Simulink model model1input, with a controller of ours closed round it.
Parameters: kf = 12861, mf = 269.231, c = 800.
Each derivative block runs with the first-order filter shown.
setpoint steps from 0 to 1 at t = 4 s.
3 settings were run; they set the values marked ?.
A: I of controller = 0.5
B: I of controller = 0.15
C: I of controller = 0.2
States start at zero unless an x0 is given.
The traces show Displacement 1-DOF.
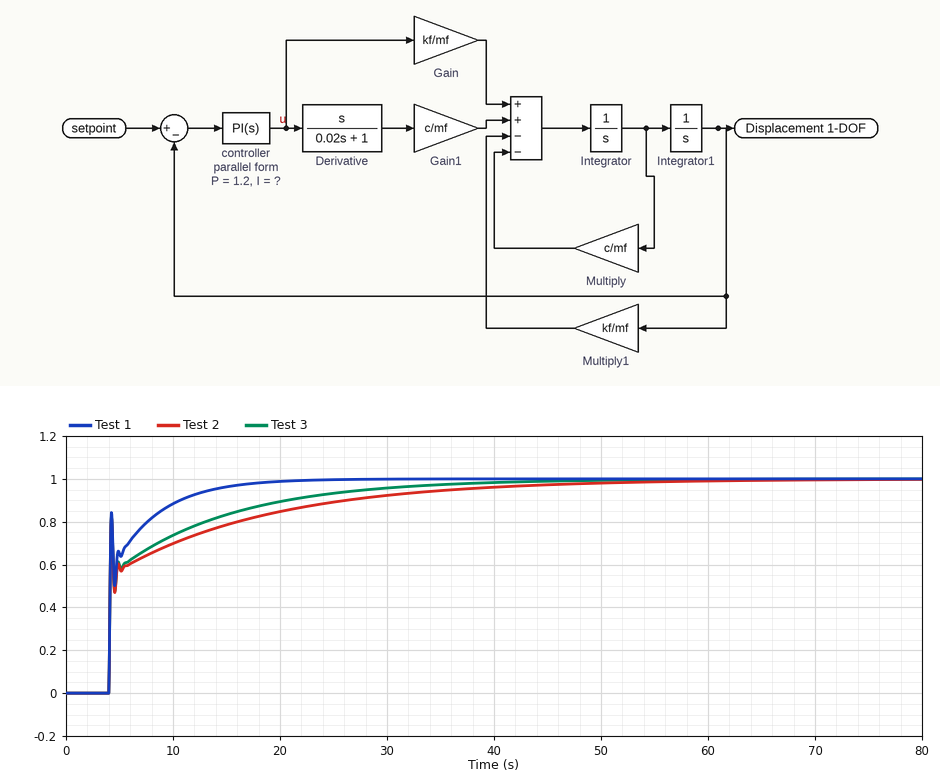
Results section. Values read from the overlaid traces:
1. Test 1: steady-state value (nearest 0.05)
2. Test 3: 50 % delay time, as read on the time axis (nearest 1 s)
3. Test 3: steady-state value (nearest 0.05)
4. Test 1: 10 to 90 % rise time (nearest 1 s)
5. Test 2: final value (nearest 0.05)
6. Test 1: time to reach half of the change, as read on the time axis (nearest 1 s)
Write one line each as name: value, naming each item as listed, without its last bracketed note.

Test 1: steady-state value: 1.00
Test 3: 50 % delay time, as read on the time axis: 4 s
Test 3: steady-state value: 1.00
Test 1: 10 to 90 % rise time: 7 s
Test 2: final value: 1.00
Test 1: time to reach half of the change, as read on the time axis: 4 s
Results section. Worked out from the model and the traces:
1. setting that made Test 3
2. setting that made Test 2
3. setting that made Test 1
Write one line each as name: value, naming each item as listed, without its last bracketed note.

setting that made Test 3: C
setting that made Test 2: B
setting that made Test 1: A
